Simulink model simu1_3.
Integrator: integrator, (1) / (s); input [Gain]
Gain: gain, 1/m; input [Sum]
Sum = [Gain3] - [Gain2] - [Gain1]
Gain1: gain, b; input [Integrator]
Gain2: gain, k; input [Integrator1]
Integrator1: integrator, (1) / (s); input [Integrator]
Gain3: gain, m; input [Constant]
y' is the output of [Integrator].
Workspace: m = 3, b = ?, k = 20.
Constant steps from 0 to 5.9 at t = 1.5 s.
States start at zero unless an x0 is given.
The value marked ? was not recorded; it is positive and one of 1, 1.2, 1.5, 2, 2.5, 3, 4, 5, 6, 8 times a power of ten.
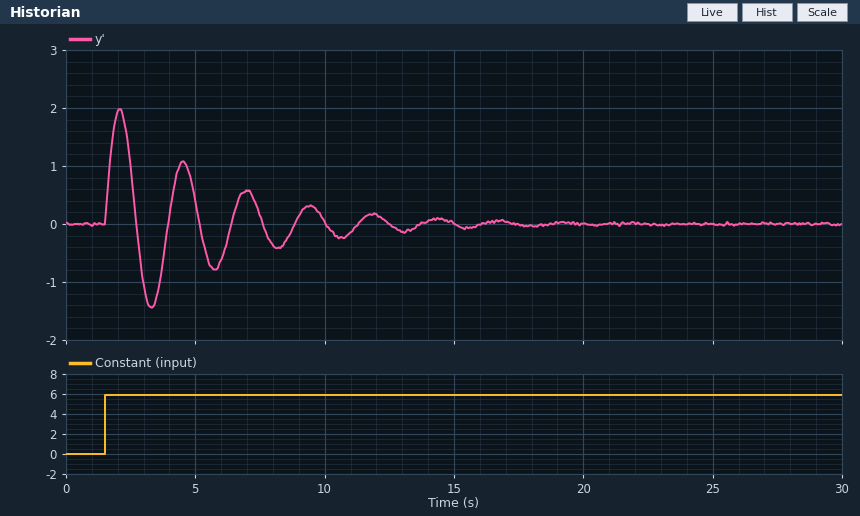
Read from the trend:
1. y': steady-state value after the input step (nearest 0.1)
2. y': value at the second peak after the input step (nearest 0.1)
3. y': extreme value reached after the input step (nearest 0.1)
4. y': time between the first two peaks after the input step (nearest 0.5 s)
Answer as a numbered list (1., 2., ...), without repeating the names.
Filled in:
1. 0.0
2. 1.1
3. 2.0
4. 2.5 s
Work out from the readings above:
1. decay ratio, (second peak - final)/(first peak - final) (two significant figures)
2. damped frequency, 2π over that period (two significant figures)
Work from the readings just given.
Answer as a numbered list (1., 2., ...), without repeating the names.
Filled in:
1. 0.55
2. 2.5 rad/s
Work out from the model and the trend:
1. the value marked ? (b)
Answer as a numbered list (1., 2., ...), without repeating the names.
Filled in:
1. 1.5
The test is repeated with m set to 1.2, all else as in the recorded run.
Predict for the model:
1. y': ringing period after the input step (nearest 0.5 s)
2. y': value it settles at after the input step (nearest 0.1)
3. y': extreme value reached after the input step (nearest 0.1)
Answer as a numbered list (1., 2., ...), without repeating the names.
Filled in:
1. 1.5 s
2. 0.0
3. 1.2
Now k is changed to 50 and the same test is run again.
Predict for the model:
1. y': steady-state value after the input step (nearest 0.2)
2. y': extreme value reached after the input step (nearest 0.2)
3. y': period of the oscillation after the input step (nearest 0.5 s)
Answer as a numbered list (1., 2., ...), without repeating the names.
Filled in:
1. 0.0
2. 1.4
3. 1.5 s
